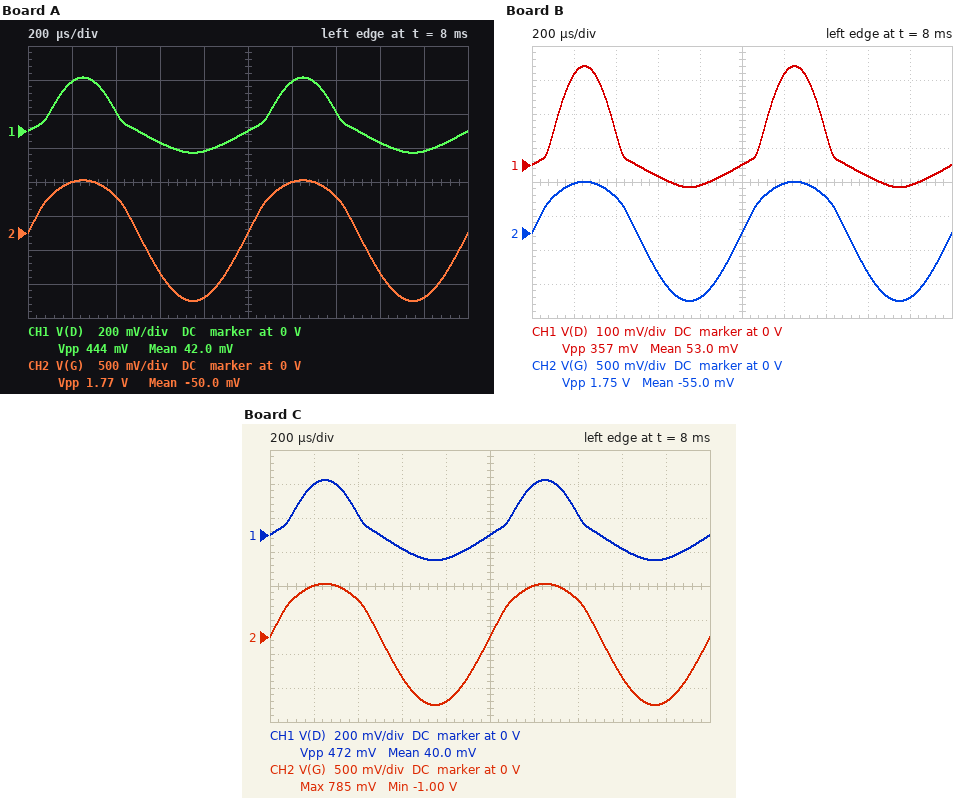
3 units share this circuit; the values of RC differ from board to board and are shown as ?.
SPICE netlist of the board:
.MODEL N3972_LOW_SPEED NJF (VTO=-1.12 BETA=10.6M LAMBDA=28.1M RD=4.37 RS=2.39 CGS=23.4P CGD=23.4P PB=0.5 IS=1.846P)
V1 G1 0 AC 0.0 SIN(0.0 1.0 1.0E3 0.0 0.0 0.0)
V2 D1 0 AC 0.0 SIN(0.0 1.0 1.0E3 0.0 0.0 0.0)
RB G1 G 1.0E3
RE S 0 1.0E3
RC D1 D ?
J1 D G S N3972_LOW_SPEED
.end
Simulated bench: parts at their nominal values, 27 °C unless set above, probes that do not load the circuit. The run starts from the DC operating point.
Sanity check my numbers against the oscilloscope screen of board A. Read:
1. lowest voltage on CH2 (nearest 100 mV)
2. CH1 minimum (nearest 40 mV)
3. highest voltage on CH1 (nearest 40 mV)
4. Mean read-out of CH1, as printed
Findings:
-1.0 V
-120 mV
320 mV
42.0 mV
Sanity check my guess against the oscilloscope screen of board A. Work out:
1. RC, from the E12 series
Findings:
8.2 kΩ
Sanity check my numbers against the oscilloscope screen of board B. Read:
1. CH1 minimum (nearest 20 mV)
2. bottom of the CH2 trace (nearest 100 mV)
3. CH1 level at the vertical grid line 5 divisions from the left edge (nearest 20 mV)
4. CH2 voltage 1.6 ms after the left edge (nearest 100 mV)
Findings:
-60 mV
-1.0 V
0 V
-600 mV
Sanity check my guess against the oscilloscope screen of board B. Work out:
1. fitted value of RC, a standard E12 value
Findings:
18 kΩ
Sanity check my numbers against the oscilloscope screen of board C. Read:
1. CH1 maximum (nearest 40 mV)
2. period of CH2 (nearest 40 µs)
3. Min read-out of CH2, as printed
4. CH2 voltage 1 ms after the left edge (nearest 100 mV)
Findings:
320 mV
1.00 ms
-1.00 V
0 V
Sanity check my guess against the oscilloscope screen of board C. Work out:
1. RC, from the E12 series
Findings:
6.8 kΩ
